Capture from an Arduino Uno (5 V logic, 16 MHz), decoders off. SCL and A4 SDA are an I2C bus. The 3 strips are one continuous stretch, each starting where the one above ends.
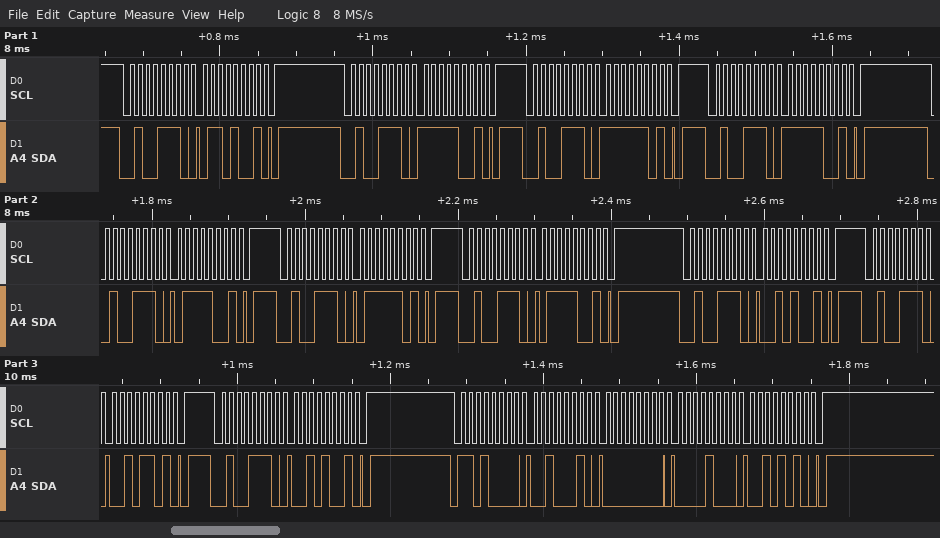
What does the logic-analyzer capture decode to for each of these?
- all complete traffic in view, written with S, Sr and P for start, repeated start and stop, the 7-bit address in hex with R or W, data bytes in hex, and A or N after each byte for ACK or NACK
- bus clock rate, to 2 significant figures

S 27W A 69 A P S 27W A F9 A P S 27W A FD A P S 27W A F9 A P S 27W A 79 A P S 27W A 7D A P S 27W A 79 A P S 27W A 29 A P S 27W A 2D A P S 27W A 29 A P S 68W A 22 A 00 A 08 A 2A A P
100 kHz
